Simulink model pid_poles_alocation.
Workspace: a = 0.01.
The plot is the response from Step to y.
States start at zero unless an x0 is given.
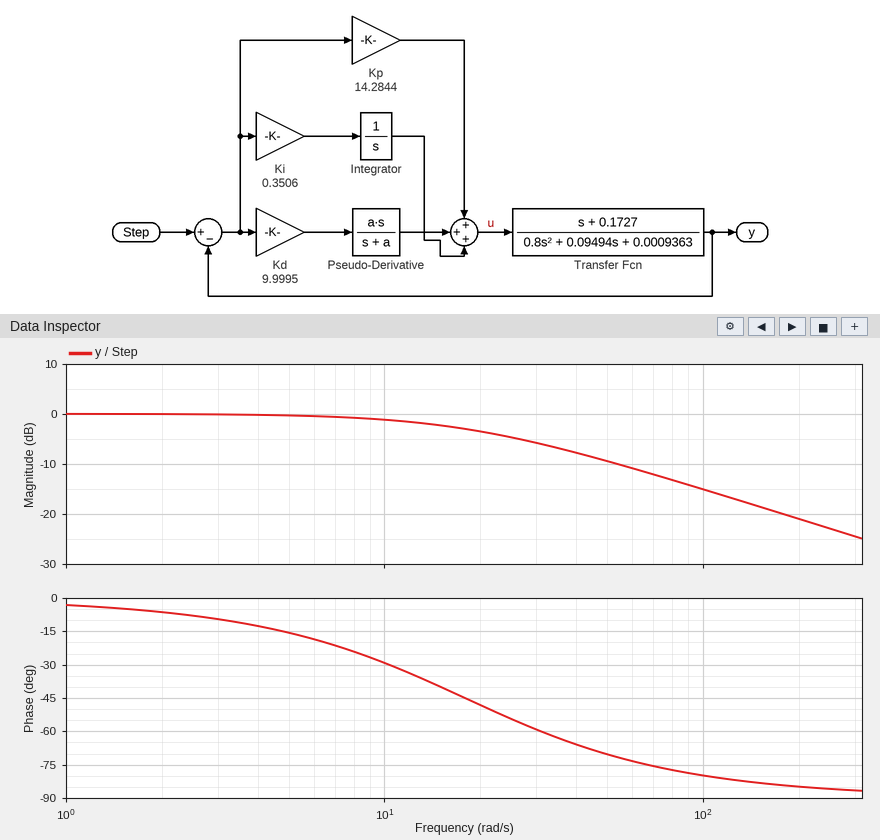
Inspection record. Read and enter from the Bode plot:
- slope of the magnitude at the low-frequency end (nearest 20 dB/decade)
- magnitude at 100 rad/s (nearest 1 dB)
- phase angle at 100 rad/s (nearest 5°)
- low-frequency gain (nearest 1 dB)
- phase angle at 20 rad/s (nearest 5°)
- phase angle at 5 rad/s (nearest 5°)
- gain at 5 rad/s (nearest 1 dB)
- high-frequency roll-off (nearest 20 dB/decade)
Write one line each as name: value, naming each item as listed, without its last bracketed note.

slope of the magnitude at the low-frequency end: 0 dB/decade
magnitude at 100 rad/s: -15 dB
phase angle at 100 rad/s: -80°
low-frequency gain: 0 dB
phase angle at 20 rad/s: -50°
phase angle at 5 rad/s: -15°
gain at 5 rad/s: 0 dB
high-frequency roll-off: -20 dB/decade
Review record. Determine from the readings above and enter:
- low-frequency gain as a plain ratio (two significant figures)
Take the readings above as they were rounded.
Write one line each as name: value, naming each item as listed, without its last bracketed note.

low-frequency gain as a plain ratio: 1.0
